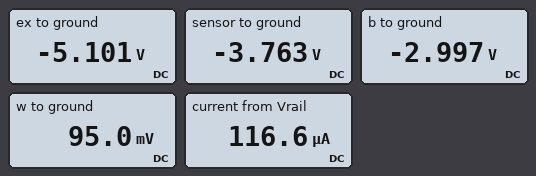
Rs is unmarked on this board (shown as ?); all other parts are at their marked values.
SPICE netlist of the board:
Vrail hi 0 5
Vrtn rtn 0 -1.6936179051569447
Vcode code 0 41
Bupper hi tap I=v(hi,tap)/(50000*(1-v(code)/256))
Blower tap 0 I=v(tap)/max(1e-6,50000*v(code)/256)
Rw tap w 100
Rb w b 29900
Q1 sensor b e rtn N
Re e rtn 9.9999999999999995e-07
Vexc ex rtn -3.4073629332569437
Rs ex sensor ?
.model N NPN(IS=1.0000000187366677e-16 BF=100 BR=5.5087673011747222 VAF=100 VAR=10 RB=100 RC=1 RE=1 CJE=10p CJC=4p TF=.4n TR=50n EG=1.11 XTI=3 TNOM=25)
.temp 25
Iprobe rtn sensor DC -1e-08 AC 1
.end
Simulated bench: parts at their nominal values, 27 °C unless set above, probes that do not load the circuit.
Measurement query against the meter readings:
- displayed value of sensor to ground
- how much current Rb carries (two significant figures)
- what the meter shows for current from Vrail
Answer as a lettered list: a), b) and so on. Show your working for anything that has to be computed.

a) -3.763 V
b) (95 mV - (-2.997 V)) / 29.9 kΩ = 100 µA
c) 116.6 µA
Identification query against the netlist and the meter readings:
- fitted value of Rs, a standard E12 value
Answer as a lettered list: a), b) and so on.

a) 1.8 kΩ
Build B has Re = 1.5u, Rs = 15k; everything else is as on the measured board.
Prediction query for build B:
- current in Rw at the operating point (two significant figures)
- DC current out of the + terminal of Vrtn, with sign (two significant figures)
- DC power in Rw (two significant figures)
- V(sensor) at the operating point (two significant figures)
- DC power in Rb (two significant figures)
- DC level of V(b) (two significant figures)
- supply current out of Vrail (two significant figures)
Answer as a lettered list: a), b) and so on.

a) 49 µA
b) -49 µA
c) 240 nW
d) -1.7 V
e) 71 µW
f) -990 mV
g) 110 µA
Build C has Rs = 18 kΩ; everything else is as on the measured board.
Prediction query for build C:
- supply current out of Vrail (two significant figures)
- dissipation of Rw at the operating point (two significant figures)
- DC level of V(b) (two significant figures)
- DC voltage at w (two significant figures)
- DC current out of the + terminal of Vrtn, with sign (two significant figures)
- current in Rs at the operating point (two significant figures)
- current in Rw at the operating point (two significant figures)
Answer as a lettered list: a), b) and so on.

a) 110 µA
b) 230 nW
c) -980 mV
d) 470 mV
e) -48 µA
f) 190 µA
g) 48 µA
